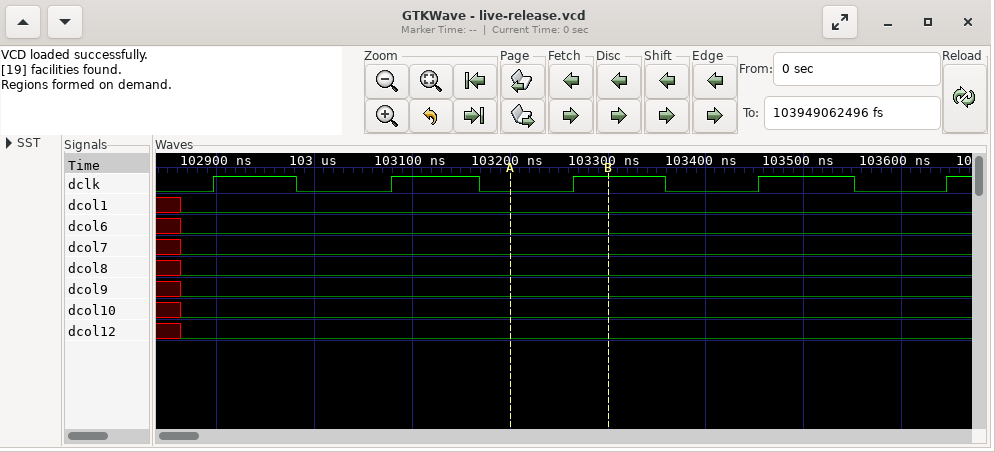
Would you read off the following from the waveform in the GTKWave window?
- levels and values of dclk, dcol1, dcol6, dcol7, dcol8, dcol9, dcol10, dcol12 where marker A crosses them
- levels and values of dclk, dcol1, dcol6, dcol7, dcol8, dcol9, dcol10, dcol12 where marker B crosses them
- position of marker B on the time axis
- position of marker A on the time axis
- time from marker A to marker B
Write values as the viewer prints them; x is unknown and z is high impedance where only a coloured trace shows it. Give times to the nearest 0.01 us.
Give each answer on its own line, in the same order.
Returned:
dclk=0, dcol1=0, dcol6=0, dcol7=0, dcol8=0, dcol9=0, dcol10=0, dcol12=0
dclk=1, dcol1=0, dcol6=0, dcol7=0, dcol8=0, dcol9=0, dcol10=0, dcol12=0
103.3 us
103.2 us
0.1 us
